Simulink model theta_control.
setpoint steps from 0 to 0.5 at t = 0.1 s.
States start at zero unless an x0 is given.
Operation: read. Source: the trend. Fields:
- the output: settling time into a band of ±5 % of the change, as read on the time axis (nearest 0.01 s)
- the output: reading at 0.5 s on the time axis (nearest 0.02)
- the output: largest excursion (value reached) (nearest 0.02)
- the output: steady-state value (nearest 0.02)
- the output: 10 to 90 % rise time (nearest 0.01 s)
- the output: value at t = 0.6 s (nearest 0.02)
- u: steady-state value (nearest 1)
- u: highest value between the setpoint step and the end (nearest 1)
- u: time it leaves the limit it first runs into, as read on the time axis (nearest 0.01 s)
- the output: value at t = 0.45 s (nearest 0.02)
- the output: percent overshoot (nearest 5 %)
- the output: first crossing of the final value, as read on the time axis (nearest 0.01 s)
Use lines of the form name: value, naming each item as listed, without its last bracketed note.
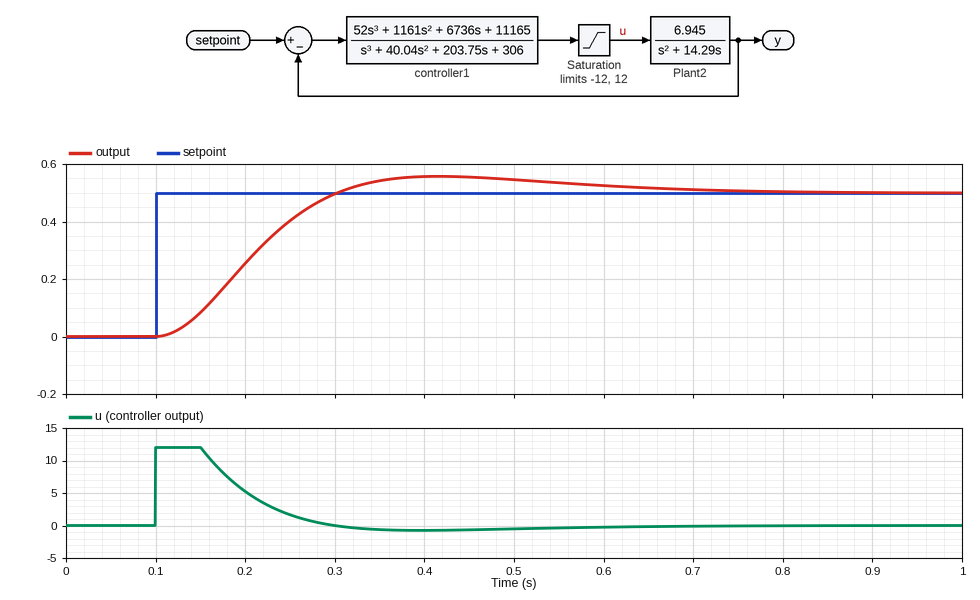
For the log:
the output: settling time into a band of ±5 % of the change, as read on the time axis: 0.60 s
the output: reading at 0.5 s on the time axis: 0.54
the output: largest excursion (value reached): 0.56
the output: steady-state value: 0.50
the output: 10 to 90 % rise time: 0.13 s
the output: value at t = 0.6 s: 0.52
u: steady-state value: 0
u: highest value between the setpoint step and the end: 12
u: time it leaves the limit it first runs into, as read on the time axis: 0.15 s
the output: value at t = 0.45 s: 0.56
the output: percent overshoot: 10 %
the output: first crossing of the final value, as read on the time axis: 0.30 s
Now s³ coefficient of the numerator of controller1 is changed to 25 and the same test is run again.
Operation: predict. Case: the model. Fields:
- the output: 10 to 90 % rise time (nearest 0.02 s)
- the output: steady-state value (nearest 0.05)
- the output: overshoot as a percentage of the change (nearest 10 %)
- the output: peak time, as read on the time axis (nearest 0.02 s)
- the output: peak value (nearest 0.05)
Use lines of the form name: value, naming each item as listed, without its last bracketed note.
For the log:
the output: 10 to 90 % rise time: 0.12 s
the output: steady-state value: 0.50
the output: overshoot as a percentage of the change: 20 %
the output: peak time, as read on the time axis: 0.36 s
the output: peak value: 0.60
